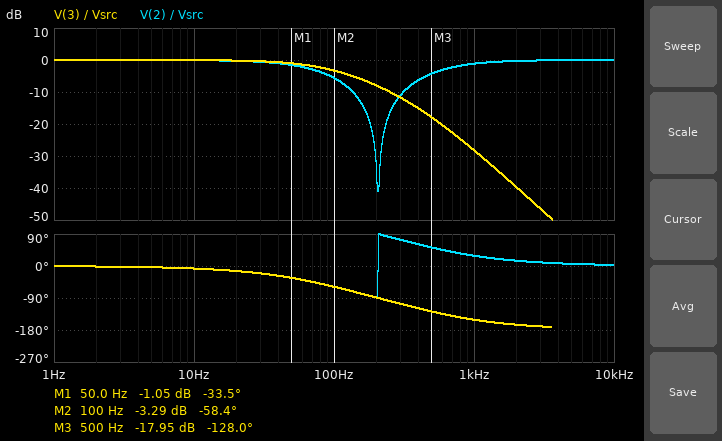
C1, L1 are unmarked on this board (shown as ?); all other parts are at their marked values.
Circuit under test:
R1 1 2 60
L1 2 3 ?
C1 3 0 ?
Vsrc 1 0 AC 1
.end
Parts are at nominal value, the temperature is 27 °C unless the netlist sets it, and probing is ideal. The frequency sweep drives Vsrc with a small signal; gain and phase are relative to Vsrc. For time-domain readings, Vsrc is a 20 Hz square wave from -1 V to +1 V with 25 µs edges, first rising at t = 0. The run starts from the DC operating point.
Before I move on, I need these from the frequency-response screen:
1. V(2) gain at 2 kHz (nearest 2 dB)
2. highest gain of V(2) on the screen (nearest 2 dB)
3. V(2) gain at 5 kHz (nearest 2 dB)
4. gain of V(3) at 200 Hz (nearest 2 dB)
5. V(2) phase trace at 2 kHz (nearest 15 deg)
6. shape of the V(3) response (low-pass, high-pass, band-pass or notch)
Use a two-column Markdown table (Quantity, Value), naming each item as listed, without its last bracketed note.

| Quantity | Value |
|---|---|
| V(2) gain at 2 kHz | 0 dB |
| highest gain of V(2) on the screen | 0 dB |
| V(2) gain at 5 kHz | 0 dB |
| gain of V(3) at 200 Hz | -8 dB |
| V(2) phase trace at 2 kHz | 15 deg |
| shape of the V(3) response | low-pass |
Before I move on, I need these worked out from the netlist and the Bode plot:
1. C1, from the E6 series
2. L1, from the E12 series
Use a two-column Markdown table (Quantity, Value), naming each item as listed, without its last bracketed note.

| Quantity | Value |
|---|---|
| C1, from the E6 series | 33 µF |
| L1, from the E12 series | 18 mH |
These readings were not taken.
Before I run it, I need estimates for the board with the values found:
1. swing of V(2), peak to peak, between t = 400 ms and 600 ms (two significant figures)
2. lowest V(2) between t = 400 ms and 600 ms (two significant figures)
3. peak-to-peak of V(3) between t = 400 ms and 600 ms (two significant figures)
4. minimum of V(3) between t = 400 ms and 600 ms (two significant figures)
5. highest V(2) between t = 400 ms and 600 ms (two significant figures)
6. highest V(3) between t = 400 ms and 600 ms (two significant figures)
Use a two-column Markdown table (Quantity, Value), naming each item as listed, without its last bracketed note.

| Quantity | Value |
|---|---|
| swing of V(2), peak to peak, between t = 400 ms and 600 ms | 2.0 V |
| lowest V(2) between t = 400 ms and 600 ms | -1.0 V |
| peak-to-peak of V(3) between t = 400 ms and 600 ms | 2.0 V |
| minimum of V(3) between t = 400 ms and 600 ms | -1.0 V |
| highest V(2) between t = 400 ms and 600 ms | 1.0 V |
| highest V(3) between t = 400 ms and 600 ms | 1.0 V |
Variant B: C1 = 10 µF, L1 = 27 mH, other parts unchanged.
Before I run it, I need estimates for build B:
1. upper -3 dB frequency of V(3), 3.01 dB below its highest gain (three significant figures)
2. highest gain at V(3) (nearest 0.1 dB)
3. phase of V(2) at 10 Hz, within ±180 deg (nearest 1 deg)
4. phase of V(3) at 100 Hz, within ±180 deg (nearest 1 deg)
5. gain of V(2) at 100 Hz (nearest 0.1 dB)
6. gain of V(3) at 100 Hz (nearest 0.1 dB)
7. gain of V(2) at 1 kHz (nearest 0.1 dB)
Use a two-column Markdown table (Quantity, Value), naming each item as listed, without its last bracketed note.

| Quantity | Value |
|---|---|
| upper -3 dB frequency of V(3), 3.01 dB below its highest gain | 346 Hz |
| highest gain at V(3) | 0.5 dB |
| phase of V(2) at 10 Hz, within ±180 deg | -2 deg |
| phase of V(3) at 100 Hz, within ±180 deg | -23 deg |
| gain of V(2) at 100 Hz | -0.7 dB |
| gain of V(3) at 100 Hz | 0.3 dB |
| gain of V(2) at 1 kHz | -0.6 dB |
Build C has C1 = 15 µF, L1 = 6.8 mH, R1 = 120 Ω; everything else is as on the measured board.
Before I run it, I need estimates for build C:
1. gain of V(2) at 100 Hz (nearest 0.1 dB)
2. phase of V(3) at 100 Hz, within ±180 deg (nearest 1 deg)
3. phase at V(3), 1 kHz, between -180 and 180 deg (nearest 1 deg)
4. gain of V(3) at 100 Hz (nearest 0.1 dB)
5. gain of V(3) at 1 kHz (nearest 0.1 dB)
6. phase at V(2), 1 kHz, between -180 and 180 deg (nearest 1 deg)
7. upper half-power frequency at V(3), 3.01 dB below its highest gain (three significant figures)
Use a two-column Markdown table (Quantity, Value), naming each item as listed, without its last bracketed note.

| Quantity | Value |
|---|---|
| gain of V(2) at 100 Hz | -3.8 dB |
| phase of V(3) at 100 Hz, within ±180 deg | -50 deg |
| phase at V(3), 1 kHz, between -180 and 180 deg | -105 deg |
| gain of V(3) at 100 Hz | -3.4 dB |
| gain of V(3) at 1 kHz | -21.4 dB |
| phase at V(2), 1 kHz, between -180 and 180 deg | 75 deg |
| upper half-power frequency at V(3), 3.01 dB below its highest gain | 91.3 Hz |
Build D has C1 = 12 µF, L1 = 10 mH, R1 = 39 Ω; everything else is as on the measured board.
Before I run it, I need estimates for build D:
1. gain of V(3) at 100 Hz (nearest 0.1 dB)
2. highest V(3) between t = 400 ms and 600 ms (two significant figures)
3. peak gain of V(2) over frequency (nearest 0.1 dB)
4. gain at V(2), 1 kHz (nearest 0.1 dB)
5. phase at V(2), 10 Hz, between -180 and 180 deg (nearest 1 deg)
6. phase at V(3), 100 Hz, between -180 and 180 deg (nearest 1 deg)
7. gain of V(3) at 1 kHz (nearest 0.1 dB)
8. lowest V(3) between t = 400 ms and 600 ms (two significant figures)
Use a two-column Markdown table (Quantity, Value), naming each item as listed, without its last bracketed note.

| Quantity | Value |
|---|---|
| gain of V(3) at 100 Hz | 0 dB |
| highest V(3) between t = 400 ms and 600 ms | 1.1 V |
| peak gain of V(2) over frequency | 0 dB |
| gain at V(2), 1 kHz | -2.1 dB |
| phase at V(2), 10 Hz, between -180 and 180 deg | -2 deg |
| phase at V(3), 100 Hz, between -180 and 180 deg | -17 deg |
| gain of V(3) at 1 kHz | -13.5 dB |
| lowest V(3) between t = 400 ms and 600 ms | -1.1 V |
